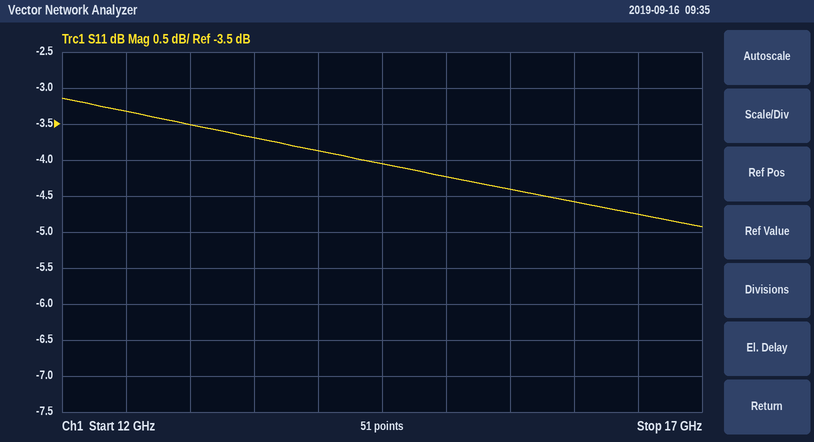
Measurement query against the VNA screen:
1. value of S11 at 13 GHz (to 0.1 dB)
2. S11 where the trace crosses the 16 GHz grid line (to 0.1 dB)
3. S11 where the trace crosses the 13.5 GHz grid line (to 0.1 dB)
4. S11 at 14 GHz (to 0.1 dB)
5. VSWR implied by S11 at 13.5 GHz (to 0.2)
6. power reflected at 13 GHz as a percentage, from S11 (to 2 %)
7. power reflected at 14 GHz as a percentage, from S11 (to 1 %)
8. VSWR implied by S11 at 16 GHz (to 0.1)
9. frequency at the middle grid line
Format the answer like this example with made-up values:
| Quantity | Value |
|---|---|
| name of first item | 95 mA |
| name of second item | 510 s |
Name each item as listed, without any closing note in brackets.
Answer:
| Quantity | Value |
|---|---|
| value of S11 at 13 GHz | -3.5 dB |
| S11 where the trace crosses the 16 GHz grid line | -4.6 dB |
| S11 where the trace crosses the 13.5 GHz grid line | -3.7 dB |
| S11 at 14 GHz | -3.9 dB |
| VSWR implied by S11 at 13.5 GHz | 4.8 |
| power reflected at 13 GHz as a percentage, from S11 | 44 % |
| power reflected at 14 GHz as a percentage, from S11 | 41 % |
| VSWR implied by S11 at 16 GHz | 3.9 |
| frequency at the middle grid line | 14.5 GHz |
